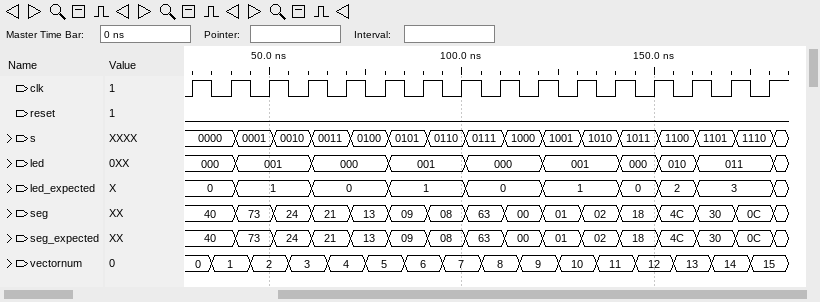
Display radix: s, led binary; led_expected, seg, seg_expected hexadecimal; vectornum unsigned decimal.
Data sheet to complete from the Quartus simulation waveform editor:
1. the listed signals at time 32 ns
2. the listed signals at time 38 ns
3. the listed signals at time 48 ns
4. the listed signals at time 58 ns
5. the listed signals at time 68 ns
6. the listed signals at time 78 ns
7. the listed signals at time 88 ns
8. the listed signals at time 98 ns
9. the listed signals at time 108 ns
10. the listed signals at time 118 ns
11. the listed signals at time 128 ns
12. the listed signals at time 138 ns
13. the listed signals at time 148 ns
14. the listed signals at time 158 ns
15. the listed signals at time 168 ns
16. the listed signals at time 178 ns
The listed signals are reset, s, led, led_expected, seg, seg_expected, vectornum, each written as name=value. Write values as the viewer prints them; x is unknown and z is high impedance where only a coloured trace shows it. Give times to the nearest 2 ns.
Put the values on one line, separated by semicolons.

reset=0, s=0000, led=000, led_expected=0, seg=40, seg_expected=40, vectornum=0; reset=0, s=0000, led=000, led_expected=0, seg=40, seg_expected=40, vectornum=1; reset=0, s=0001, led=001, led_expected=1, seg=73, seg_expected=73, vectornum=2; reset=0, s=0010, led=001, led_expected=1, seg=24, seg_expected=24, vectornum=3; reset=0, s=0011, led=000, led_expected=0, seg=21, seg_expected=21, vectornum=4; reset=0, s=0100, led=000, led_expected=0, seg=13, seg_expected=13, vectornum=5; reset=0, s=0101, led=001, led_expected=1, seg=09, seg_expected=09, vectornum=6; reset=0, s=0110, led=001, led_expected=1, seg=08, seg_expected=08, vectornum=7; reset=0, s=0111, led=000, led_expected=0, seg=63, seg_expected=63, vectornum=8; reset=0, s=1000, led=000, led_expected=0, seg=00, seg_expected=00, vectornum=9; reset=0, s=1001, led=001, led_expected=1, seg=01, seg_expected=01, vectornum=10; reset=0, s=1010, led=001, led_expected=1, seg=02, seg_expected=02, vectornum=11; reset=0, s=1011, led=000, led_expected=0, seg=18, seg_expected=18, vectornum=12; reset=0, s=1100, led=010, led_expected=2, seg=4C, seg_expected=4C, vectornum=13; reset=0, s=1101, led=011, led_expected=3, seg=30, seg_expected=30, vectornum=14; reset=0, s=1110, led=011, led_expected=3, seg=0C, seg_expected=0C, vectornum=15
